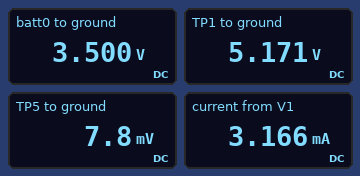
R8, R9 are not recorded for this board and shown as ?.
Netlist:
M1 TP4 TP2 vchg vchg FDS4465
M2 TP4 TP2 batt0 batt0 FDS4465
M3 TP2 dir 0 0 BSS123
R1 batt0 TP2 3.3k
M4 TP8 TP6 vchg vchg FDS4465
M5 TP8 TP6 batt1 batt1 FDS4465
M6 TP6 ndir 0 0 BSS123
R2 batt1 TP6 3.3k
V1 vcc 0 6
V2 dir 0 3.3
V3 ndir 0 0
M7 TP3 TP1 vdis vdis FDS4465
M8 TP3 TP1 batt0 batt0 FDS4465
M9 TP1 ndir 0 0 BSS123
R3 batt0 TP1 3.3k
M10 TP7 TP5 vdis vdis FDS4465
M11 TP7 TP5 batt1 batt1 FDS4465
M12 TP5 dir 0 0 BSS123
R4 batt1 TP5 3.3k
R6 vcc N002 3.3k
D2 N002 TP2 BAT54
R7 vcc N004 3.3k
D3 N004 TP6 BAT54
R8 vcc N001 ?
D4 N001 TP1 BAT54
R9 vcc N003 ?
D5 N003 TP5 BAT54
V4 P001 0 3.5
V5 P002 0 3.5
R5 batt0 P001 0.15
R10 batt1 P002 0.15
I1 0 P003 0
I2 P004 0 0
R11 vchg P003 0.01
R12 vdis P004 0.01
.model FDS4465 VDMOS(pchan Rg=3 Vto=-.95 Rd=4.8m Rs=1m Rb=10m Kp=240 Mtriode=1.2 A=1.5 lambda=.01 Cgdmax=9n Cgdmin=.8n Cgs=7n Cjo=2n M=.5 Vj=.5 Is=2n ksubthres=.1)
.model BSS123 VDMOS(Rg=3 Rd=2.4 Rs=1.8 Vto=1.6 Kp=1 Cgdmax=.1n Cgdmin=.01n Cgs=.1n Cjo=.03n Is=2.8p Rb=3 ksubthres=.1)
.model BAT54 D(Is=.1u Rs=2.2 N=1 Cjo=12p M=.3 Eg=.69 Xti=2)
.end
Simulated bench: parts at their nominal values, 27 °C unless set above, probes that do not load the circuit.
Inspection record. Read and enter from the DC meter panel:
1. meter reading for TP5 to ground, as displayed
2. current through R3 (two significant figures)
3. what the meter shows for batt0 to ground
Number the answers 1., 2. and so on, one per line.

1. 7.8 mV
2. 510 µA
3. 3.500 V
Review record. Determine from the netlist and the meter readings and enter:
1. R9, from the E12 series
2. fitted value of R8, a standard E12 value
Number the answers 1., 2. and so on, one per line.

1. 10 kΩ
2. 1.2 kΩ
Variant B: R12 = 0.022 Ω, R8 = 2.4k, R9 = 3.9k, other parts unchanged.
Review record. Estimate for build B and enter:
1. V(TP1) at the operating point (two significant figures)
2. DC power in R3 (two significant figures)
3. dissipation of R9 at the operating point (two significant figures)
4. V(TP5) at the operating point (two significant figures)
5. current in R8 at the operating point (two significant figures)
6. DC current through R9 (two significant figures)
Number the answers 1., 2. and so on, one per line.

1. 4.8 V
2. 530 µW
3. 8.4 mW
4. 12 mV
5. 400 µA
6. 1.5 mA
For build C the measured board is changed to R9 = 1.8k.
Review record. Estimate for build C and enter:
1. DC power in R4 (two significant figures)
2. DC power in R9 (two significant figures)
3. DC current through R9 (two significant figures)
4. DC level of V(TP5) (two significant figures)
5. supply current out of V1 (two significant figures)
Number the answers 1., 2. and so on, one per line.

1. 3.7 mW
2. 18 mW
3. 3.2 mA
4. 20 mV
5. 5.8 mA
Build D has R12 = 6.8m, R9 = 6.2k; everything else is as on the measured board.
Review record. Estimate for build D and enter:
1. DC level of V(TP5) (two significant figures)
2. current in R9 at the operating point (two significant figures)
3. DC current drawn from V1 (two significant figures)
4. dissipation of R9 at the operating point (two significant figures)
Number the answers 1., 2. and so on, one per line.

1. 9.5 mV
2. 930 µA
3. 3.5 mA
4. 5.3 mW
